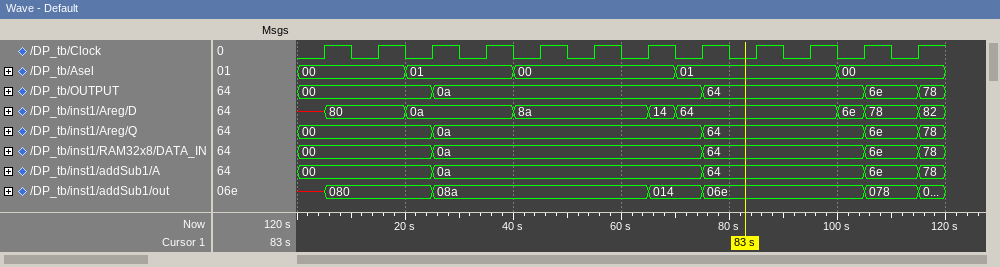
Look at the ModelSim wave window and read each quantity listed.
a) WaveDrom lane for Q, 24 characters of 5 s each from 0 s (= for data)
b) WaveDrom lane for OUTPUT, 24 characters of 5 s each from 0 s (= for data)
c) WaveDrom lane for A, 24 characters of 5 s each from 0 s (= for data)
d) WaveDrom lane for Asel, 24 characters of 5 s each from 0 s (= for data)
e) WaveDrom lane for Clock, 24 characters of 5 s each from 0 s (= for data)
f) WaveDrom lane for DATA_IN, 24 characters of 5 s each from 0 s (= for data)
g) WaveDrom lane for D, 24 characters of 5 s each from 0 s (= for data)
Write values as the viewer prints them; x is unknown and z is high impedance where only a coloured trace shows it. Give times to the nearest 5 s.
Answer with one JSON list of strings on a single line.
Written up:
["{name: 'Q', wave: '=....=.........=.....=.=', data: '00 0a 64 6e 78'}", "{name: 'OUTPUT', wave: '=....=.........=.....=.=', data: '00 0a 64 6e 78'}", "{name: 'A', wave: '=....=.........=.....=.=', data: '00 0a 64 6e 78'}", "{name: 'Asel', wave: '=...=...=.....=.....=...', data: '00 01 00 01 00'}", "{name: 'Clock', wave: '010101010101010101010101'}", "{name: 'DATA_IN', wave: '=....=.........=.....=.=', data: '00 0a 64 6e 78'}", "{name: 'D', wave: 'x=..=...=....==.....==.=', data: '80 0a 8a 14 64 6e 78 82'}"]
